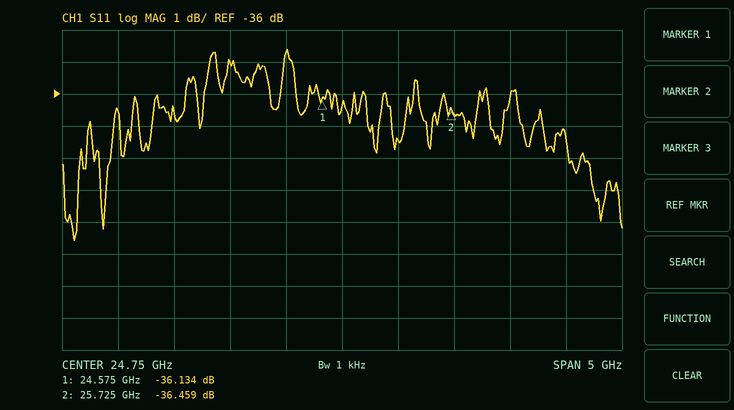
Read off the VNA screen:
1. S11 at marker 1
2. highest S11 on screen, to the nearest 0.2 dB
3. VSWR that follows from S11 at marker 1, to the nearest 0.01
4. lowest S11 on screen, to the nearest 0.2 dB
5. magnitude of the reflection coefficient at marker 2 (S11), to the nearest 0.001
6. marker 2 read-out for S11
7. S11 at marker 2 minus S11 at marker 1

-36.134 dB
-34.6 dB
1.03
-40.6 dB
0.015
-36.459 dB
-0.325 dB
